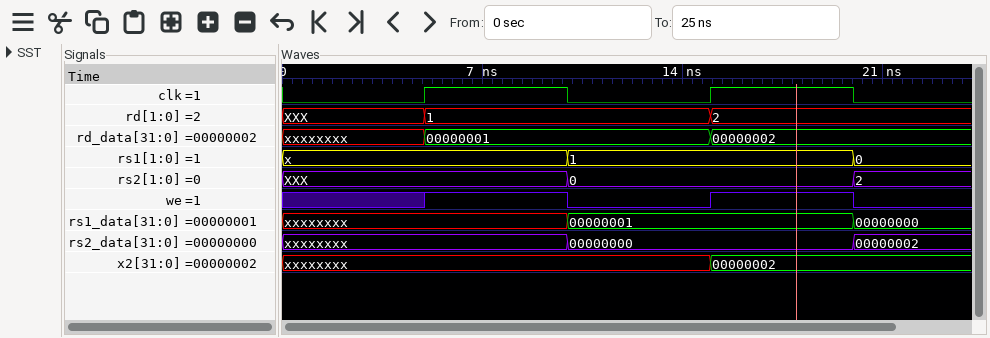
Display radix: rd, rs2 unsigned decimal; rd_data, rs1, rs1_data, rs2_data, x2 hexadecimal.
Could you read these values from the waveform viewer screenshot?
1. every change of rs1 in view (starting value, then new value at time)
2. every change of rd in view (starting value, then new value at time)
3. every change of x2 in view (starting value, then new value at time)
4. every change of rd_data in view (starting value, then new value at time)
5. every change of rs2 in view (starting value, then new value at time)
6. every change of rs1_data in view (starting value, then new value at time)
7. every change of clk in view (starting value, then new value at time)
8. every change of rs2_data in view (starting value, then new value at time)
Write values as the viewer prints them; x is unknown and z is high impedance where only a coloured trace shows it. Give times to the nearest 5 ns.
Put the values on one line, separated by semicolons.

x, 1 at 10 ns, 0 at 20 ns; XXX, 1 at 5 ns, 2 at 15 ns; xxxxxxxx, 00000002 at 15 ns; xxxxxxxx, 00000001 at 5 ns, 00000002 at 15 ns; XXX, 0 at 10 ns, 2 at 20 ns; xxxxxxxx, 00000001 at 10 ns, 00000000 at 20 ns; 0, 1 at 5 ns, 0 at 10 ns, 1 at 15 ns, 0 at 20 ns; xxxxxxxx, 00000000 at 10 ns, 00000002 at 20 ns
